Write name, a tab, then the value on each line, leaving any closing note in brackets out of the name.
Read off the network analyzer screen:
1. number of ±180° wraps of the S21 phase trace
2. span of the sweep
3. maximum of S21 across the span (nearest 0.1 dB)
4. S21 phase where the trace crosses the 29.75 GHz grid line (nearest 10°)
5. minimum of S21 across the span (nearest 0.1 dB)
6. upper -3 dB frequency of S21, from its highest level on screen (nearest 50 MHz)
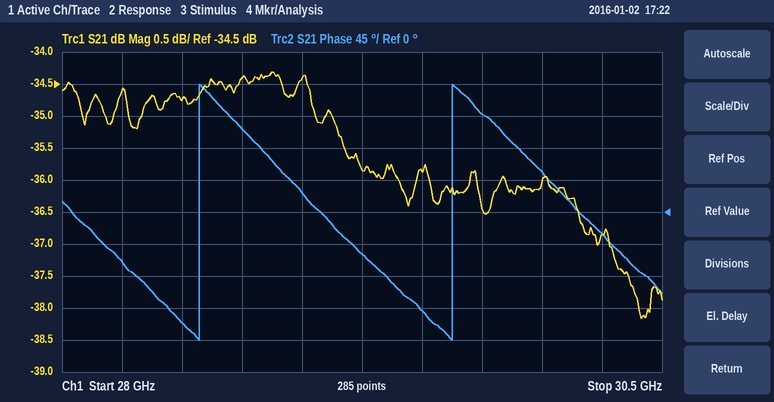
number of ±180° wraps of the S21 phase trace	2
span of the sweep	2.5 GHz
maximum of S21 across the span	-34.3 dB
S21 phase where the trace crosses the 29.75 GHz grid line	140°
minimum of S21 across the span	-38.2 dB
upper -3 dB frequency of S21, from its highest level on screen	30.30 GHz
